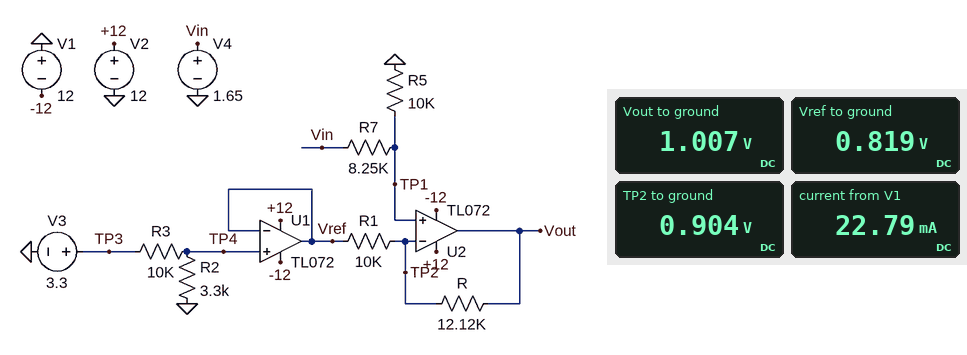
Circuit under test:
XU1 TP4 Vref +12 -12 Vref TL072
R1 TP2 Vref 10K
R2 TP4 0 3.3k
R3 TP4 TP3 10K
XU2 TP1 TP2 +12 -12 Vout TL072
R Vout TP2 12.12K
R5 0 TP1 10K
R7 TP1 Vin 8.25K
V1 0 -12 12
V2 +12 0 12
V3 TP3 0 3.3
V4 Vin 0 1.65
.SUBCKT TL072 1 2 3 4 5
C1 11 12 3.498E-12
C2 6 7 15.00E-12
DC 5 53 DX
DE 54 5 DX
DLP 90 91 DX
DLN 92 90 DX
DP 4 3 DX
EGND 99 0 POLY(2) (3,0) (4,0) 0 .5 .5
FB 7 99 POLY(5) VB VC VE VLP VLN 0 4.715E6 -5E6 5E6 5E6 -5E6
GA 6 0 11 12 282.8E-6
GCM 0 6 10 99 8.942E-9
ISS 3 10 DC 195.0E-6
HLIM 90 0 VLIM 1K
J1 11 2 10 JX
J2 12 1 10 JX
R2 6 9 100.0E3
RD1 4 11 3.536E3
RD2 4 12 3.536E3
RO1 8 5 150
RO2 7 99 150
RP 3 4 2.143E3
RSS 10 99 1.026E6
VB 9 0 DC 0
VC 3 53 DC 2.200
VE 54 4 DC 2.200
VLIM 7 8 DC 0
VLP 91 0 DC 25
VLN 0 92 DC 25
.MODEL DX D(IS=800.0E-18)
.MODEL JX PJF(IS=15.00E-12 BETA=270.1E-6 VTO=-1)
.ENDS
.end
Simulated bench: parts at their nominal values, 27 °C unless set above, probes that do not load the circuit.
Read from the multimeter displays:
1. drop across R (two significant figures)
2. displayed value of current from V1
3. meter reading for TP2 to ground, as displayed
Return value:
100 mV
22.79 mA
0.904 V
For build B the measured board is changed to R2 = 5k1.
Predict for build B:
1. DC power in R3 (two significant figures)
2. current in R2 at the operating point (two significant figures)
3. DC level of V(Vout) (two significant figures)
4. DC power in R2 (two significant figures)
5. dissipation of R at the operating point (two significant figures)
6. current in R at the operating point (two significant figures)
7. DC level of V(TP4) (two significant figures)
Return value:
480 µW
220 µA
650 mV
240 µW
5.4 µW
21 µA
1.1 V
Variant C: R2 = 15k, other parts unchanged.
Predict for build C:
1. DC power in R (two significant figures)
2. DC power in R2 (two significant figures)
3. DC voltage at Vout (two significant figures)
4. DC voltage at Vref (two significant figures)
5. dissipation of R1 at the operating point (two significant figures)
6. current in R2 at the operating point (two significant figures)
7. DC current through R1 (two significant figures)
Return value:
140 µW
260 µW
-400 mV
2.0 V
120 µW
130 µA
110 µA
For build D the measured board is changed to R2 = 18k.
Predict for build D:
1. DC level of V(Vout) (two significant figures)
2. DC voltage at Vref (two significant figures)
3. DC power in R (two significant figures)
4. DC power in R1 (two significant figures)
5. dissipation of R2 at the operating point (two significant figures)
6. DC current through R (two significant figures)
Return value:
-570 mV
2.1 V
180 µW
150 µW
250 µW
120 µA
